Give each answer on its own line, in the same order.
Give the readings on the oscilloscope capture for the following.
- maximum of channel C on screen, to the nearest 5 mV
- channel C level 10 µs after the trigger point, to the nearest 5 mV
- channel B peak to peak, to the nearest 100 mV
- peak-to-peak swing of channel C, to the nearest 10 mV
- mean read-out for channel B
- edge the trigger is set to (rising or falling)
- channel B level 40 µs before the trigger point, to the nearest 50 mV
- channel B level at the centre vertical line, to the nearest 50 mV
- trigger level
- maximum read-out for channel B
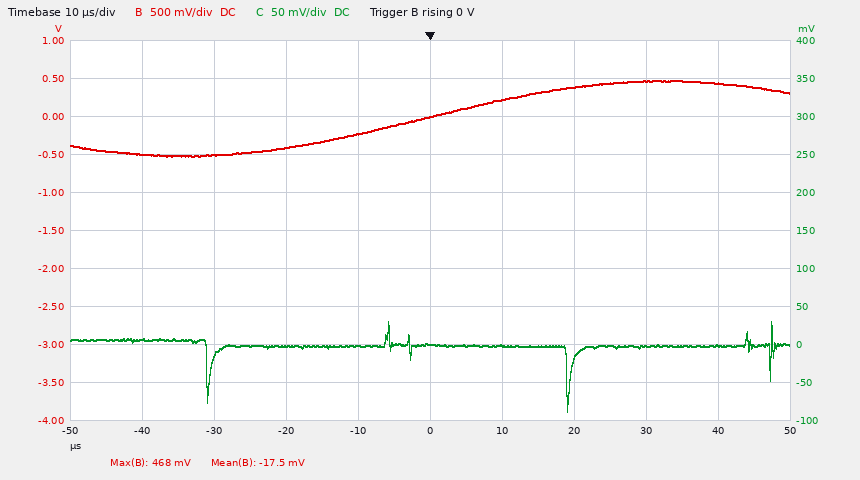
30 mV
0 mV
1.00 V
120 mV
-17.5 mV
rising
-500 mV
0 mV
0 V
468 mV
